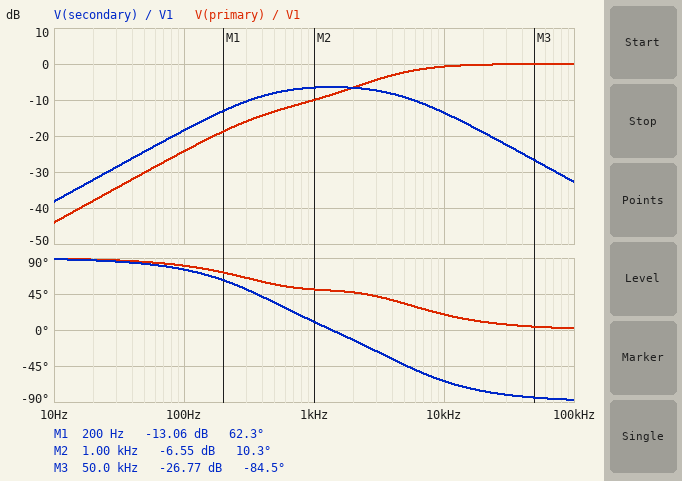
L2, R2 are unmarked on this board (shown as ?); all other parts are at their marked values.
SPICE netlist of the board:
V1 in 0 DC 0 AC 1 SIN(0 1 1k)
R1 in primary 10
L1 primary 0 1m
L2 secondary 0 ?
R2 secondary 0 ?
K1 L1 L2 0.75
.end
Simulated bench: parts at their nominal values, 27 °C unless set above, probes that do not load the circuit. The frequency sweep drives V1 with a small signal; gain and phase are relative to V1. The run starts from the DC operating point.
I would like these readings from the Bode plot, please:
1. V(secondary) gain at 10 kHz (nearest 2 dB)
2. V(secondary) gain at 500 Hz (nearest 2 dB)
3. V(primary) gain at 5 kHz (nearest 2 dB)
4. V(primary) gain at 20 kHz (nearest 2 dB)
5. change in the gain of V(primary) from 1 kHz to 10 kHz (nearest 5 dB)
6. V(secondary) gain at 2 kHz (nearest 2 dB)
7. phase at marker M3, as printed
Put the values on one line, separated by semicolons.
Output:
-14 dB; -8 dB; -2 dB; 0 dB; 10 dB; -6 dB; -84.5 deg
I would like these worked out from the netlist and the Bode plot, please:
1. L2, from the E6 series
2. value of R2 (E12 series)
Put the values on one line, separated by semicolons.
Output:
6.8 mH; 22 Ω
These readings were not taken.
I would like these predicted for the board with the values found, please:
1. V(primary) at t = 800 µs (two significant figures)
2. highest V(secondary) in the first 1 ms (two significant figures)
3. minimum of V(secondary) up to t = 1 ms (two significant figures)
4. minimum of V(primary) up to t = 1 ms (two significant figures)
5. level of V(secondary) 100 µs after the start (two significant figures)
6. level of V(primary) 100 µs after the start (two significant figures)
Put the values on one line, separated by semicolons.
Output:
-120 mV; 360 mV; -500 mV; -330 mV; 190 mV; 250 mV
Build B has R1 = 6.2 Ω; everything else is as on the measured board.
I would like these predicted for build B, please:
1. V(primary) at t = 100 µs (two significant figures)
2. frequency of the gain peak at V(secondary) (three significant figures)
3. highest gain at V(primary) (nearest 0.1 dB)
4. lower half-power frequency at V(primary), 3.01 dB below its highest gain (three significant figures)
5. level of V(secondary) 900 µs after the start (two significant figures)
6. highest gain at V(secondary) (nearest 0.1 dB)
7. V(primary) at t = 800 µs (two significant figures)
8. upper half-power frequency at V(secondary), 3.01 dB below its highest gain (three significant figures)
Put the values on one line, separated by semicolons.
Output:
330 mV; 1.08 kHz; 0 dB; 2.62 kHz; -400 mV; -3.5 dB; -230 mV; 3.74 kHz
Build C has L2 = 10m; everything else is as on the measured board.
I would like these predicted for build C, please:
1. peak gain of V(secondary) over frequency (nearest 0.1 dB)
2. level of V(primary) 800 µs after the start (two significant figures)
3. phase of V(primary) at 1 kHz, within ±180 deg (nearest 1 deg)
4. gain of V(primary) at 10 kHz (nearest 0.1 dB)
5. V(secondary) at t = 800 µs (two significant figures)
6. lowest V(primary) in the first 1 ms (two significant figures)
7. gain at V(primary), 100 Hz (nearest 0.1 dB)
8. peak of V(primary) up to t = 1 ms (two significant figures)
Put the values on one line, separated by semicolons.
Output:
-7.4 dB; -93 mV; 55 deg; -0.7 dB; -430 mV; -300 mV; -24.4 dB; 250 mV
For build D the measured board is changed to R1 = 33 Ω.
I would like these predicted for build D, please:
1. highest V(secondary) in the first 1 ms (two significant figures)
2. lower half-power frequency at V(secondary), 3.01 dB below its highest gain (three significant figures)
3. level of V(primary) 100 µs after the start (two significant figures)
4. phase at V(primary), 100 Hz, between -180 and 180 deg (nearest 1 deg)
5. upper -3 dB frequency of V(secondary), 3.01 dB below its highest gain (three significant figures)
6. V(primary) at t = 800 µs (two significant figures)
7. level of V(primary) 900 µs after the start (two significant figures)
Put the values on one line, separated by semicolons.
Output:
120 mV; 453 Hz; 92 mV; 83 deg; 13.6 kHz; -21 mV; 46 mV
